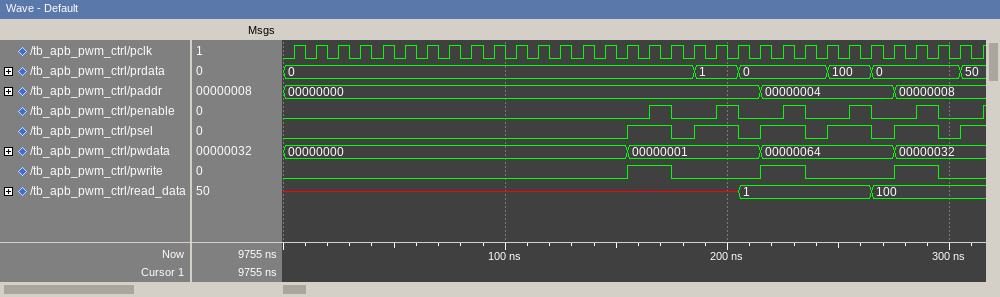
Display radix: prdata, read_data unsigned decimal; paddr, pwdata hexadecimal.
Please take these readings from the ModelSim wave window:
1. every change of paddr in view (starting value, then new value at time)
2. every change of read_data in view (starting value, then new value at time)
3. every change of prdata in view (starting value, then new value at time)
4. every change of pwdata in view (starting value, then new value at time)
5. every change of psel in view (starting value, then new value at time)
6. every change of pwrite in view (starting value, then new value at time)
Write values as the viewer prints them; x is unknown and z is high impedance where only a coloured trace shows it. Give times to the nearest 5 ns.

00000000, 00000004 at 215 ns, 00000008 at 275 ns
x, 1 at 205 ns, 100 at 265 ns
0, 1 at 185 ns, 0 at 205 ns, 100 at 245 ns, 0 at 265 ns, 50 at 305 ns
00000000, 00000001 at 155 ns, 00000064 at 215 ns, 00000032 at 275 ns
0, 1 at 155 ns, 0 at 175 ns, 1 at 185 ns, 0 at 205 ns, 1 at 215 ns, 0 at 235 ns, 1 at 245 ns, 0 at 265 ns, 1 at 275 ns, 0 at 295 ns, 1 at 305 ns
0, 1 at 155 ns, 0 at 175 ns, 1 at 215 ns, 0 at 235 ns, 1 at 275 ns, 0 at 295 ns
